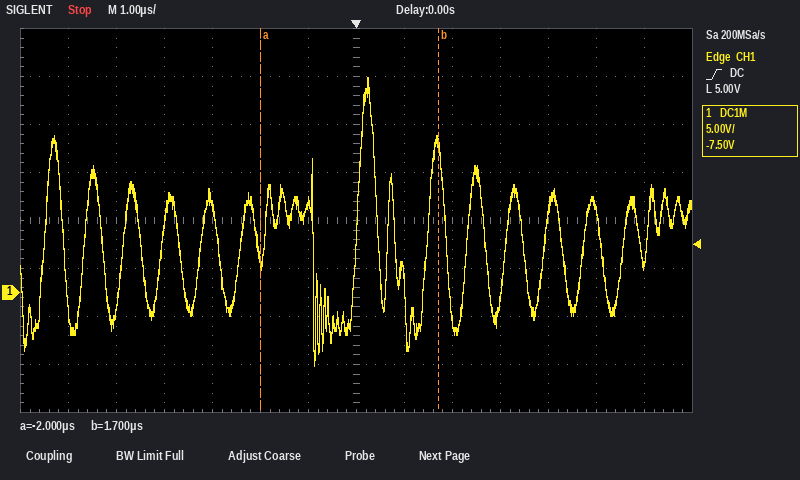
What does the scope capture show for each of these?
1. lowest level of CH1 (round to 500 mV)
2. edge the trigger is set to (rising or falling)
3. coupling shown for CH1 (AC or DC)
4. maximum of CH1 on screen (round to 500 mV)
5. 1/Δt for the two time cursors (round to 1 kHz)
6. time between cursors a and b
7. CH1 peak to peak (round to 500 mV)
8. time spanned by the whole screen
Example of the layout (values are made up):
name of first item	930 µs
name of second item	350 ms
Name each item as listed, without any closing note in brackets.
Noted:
lowest level of CH1	-7.5 V
edge the trigger is set to	rising
coupling shown for CH1	DC
maximum of CH1 on screen	22.5 V
1/Δt for the two time cursors	270 kHz
time between cursors a and b	3.7 µs
CH1 peak to peak	30.0 V
time spanned by the whole screen	14 µs
